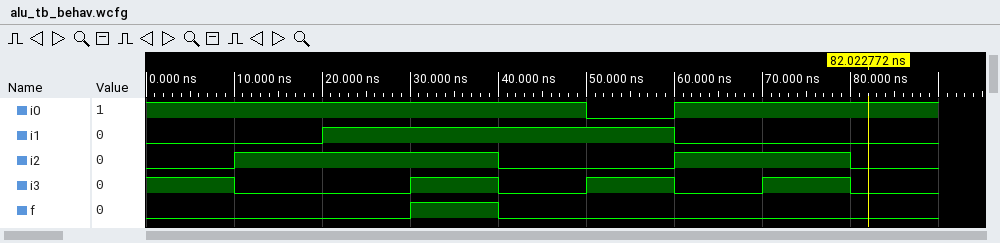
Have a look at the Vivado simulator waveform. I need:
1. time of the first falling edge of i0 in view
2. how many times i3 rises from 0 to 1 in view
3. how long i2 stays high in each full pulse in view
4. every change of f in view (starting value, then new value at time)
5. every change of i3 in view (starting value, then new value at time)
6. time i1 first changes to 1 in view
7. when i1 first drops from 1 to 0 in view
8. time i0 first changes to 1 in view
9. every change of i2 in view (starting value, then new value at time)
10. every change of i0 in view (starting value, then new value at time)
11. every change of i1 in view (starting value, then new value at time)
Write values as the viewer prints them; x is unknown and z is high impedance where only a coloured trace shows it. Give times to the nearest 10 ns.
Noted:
50 ns
3
30 ns, 20 ns
0, 1 at 30 ns, 0 at 40 ns
1, 0 at 10 ns, 1 at 30 ns, 0 at 40 ns, 1 at 50 ns, 0 at 60 ns, 1 at 70 ns, 0 at 80 ns
20 ns
60 ns
60 ns
0, 1 at 10 ns, 0 at 40 ns, 1 at 60 ns, 0 at 80 ns
1, 0 at 50 ns, 1 at 60 ns
0, 1 at 20 ns, 0 at 60 ns
